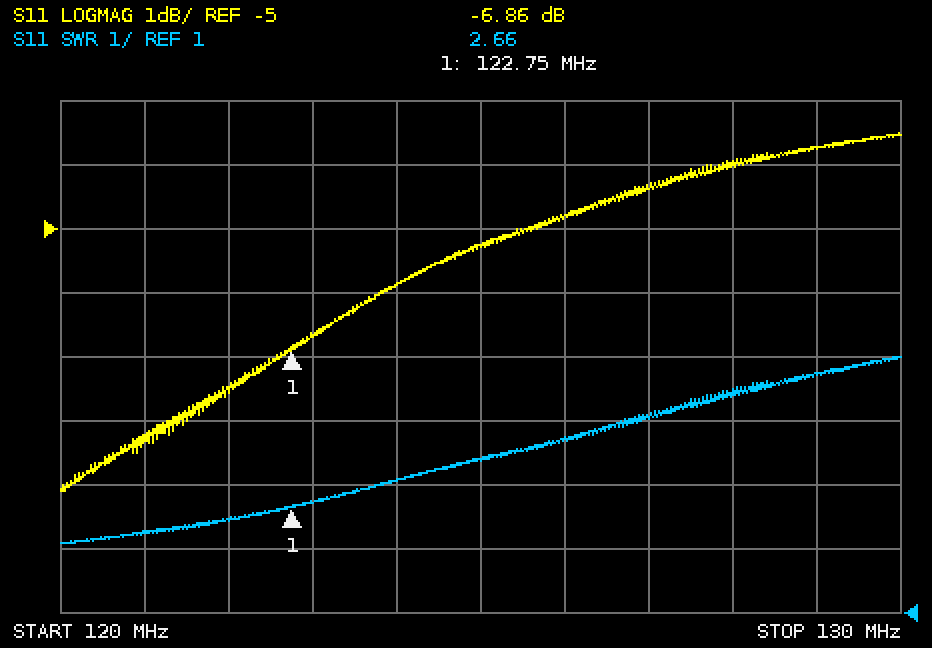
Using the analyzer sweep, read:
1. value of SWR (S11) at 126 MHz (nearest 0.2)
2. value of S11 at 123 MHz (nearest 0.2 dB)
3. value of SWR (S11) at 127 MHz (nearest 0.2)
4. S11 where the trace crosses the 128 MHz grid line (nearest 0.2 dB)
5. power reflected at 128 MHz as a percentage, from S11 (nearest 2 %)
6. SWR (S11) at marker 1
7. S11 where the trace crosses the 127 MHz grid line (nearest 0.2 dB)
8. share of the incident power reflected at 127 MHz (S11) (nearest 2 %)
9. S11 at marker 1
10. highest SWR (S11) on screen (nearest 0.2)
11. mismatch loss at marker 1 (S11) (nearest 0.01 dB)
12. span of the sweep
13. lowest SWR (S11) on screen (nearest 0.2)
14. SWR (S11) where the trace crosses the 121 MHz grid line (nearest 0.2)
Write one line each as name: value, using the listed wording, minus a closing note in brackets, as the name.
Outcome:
value of SWR (S11) at 126 MHz: 3.8
value of S11 at 123 MHz: -6.6 dB
value of SWR (S11) at 127 MHz: 4.0
S11 where the trace crosses the 128 MHz grid line: -4.0 dB
power reflected at 128 MHz as a percentage, from S11: 40 %
SWR (S11) at marker 1: 2.66
S11 where the trace crosses the 127 MHz grid line: -4.4 dB
share of the incident power reflected at 127 MHz (S11): 36 %
S11 at marker 1: -6.86 dB
highest SWR (S11) on screen: 5.0
mismatch loss at marker 1 (S11): 1.00 dB
span of the sweep: 10 MHz
lowest SWR (S11) on screen: 2.0
SWR (S11) where the trace crosses the 121 MHz grid line: 2.2
